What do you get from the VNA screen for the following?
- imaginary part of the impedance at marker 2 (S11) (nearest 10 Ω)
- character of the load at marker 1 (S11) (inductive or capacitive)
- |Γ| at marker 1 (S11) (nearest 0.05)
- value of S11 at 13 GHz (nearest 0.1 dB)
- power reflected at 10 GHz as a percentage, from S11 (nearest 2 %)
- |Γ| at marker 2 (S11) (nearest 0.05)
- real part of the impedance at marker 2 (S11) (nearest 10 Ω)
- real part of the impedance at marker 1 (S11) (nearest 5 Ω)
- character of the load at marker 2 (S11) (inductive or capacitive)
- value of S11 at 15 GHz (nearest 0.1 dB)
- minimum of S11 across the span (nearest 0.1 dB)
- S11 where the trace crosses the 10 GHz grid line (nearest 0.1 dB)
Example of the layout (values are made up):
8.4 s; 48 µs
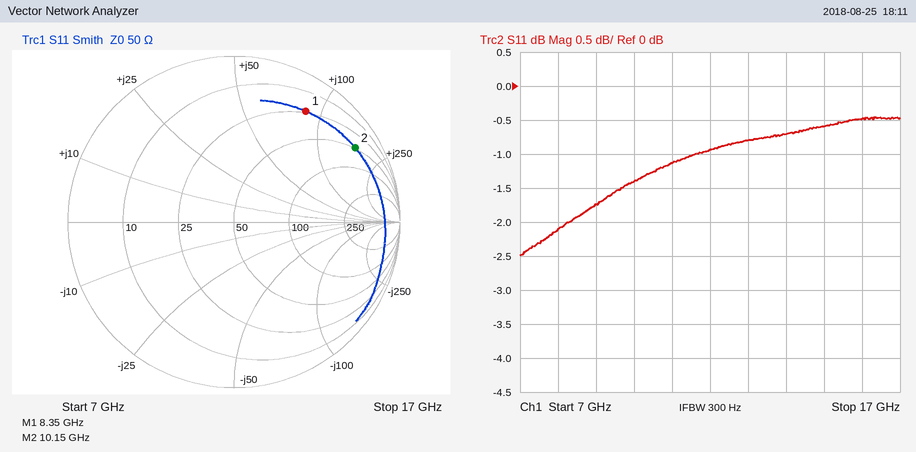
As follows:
+160 Ω; inductive; 0.80; -0.8 dB; 72 %; 0.85; 50 Ω; 25 Ω; inductive; -0.6 dB; -2.5 dB; -1.4 dB
